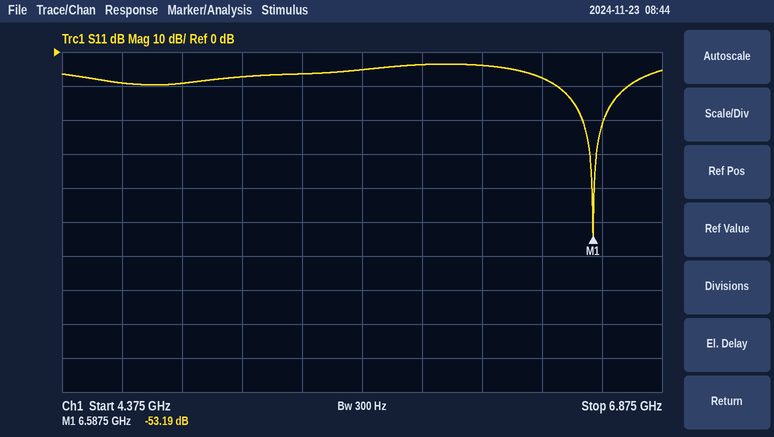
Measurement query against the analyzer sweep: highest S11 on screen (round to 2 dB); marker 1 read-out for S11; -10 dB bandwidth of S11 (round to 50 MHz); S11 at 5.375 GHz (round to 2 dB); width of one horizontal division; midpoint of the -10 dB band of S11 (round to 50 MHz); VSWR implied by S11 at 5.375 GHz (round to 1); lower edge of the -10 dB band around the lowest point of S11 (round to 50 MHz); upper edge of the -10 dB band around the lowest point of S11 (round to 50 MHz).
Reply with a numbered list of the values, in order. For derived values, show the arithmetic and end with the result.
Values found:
1. -4 dB
2. -53.19 dB
3. 6.75 GHz − 6.45 GHz = 300 MHz
4. -6 dB
5. 250 MHz
6. 6.60 GHz
7. |Γ| = 10^(-6/20) = 0.5012; VSWR = (1 + 0.5012)/(1 − 0.5012) ≈ 3
8. 6.45 GHz
9. 6.75 GHz
